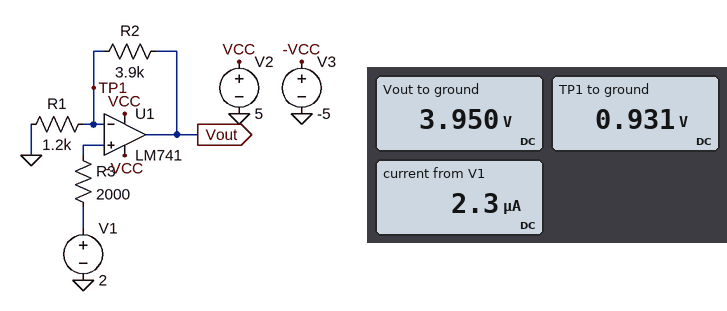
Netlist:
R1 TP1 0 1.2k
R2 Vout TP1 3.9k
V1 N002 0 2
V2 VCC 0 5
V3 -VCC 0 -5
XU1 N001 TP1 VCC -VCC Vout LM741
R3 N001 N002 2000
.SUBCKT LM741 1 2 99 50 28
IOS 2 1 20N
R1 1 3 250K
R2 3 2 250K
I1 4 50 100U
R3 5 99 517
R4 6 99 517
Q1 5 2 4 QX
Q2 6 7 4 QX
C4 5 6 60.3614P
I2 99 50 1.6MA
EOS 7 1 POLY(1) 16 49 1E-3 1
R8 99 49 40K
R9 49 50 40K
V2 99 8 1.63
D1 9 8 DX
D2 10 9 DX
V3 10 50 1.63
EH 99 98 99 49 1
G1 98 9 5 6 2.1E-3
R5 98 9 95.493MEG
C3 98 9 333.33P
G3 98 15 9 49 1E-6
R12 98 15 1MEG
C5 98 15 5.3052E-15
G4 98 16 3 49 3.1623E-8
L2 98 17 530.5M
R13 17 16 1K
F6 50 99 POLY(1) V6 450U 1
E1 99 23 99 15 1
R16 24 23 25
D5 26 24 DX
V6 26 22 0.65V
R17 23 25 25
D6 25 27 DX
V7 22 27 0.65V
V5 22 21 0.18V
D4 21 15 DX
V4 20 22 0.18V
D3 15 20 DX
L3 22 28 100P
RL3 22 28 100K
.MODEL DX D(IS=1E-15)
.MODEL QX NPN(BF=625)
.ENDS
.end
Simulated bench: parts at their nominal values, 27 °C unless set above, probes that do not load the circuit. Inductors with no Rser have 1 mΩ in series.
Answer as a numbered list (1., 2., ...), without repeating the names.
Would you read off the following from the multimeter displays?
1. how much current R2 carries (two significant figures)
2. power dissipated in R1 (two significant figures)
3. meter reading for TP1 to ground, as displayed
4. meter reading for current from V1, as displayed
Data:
1. 770 µA
2. 720 µW
3. 0.931 V
4. 2.3 µA
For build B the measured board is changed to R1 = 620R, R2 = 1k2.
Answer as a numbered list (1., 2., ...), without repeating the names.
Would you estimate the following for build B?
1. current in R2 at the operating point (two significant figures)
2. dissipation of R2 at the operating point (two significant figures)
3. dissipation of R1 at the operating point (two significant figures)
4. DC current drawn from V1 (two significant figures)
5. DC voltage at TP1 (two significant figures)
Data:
1. 2.1 mA
2. 5.5 mW
3. 2.8 mW
4. 1.5 µA
5. 1.3 V
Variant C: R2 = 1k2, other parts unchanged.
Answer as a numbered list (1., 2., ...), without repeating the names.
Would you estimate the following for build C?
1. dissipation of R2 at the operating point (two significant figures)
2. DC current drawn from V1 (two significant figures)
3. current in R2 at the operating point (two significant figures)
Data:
1. 3.2 mW
2. 220 nA
3. 1.6 mA
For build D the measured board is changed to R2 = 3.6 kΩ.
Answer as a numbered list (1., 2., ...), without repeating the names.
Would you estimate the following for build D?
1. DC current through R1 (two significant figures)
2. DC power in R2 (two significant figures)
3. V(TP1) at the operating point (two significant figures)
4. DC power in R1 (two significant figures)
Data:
1. 820 µA
2. 2.4 mW
3. 990 mV
4. 810 µW
